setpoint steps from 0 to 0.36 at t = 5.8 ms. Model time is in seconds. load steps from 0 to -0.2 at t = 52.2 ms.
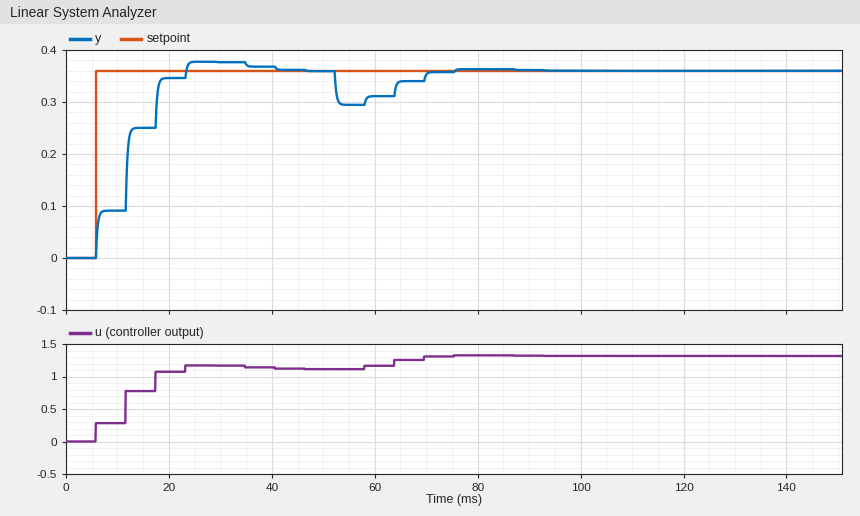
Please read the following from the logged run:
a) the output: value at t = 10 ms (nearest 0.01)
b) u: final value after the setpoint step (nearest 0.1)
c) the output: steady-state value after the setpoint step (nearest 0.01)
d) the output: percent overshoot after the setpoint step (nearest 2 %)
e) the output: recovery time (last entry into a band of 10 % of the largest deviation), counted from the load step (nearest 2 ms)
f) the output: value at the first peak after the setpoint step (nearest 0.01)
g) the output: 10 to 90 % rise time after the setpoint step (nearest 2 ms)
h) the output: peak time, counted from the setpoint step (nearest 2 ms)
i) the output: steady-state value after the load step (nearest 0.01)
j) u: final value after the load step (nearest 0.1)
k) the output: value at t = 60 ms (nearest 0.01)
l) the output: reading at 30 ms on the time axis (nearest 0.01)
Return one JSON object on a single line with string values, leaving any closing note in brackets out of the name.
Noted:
{"the output: value at t = 10 ms": "0.09", "u: final value after the setpoint step": "1.1", "the output: steady-state value after the setpoint step": "0.36", "the output: percent overshoot after the setpoint step": "4 %", "the output: recovery time (last entry into a band of 10 % of the largest deviation), counted from the load step": "18 ms", "the output: value at the first peak after the setpoint step": "0.38", "the output: 10 to 90 % rise time after the setpoint step": "12 ms", "the output: peak time, counted from the setpoint step": "24 ms", "the output: steady-state value after the load step": "0.36", "u: final value after the load step": "1.3", "the output: value at t = 60 ms": "0.31", "the output: reading at 30 ms on the time axis": "0.38"}
